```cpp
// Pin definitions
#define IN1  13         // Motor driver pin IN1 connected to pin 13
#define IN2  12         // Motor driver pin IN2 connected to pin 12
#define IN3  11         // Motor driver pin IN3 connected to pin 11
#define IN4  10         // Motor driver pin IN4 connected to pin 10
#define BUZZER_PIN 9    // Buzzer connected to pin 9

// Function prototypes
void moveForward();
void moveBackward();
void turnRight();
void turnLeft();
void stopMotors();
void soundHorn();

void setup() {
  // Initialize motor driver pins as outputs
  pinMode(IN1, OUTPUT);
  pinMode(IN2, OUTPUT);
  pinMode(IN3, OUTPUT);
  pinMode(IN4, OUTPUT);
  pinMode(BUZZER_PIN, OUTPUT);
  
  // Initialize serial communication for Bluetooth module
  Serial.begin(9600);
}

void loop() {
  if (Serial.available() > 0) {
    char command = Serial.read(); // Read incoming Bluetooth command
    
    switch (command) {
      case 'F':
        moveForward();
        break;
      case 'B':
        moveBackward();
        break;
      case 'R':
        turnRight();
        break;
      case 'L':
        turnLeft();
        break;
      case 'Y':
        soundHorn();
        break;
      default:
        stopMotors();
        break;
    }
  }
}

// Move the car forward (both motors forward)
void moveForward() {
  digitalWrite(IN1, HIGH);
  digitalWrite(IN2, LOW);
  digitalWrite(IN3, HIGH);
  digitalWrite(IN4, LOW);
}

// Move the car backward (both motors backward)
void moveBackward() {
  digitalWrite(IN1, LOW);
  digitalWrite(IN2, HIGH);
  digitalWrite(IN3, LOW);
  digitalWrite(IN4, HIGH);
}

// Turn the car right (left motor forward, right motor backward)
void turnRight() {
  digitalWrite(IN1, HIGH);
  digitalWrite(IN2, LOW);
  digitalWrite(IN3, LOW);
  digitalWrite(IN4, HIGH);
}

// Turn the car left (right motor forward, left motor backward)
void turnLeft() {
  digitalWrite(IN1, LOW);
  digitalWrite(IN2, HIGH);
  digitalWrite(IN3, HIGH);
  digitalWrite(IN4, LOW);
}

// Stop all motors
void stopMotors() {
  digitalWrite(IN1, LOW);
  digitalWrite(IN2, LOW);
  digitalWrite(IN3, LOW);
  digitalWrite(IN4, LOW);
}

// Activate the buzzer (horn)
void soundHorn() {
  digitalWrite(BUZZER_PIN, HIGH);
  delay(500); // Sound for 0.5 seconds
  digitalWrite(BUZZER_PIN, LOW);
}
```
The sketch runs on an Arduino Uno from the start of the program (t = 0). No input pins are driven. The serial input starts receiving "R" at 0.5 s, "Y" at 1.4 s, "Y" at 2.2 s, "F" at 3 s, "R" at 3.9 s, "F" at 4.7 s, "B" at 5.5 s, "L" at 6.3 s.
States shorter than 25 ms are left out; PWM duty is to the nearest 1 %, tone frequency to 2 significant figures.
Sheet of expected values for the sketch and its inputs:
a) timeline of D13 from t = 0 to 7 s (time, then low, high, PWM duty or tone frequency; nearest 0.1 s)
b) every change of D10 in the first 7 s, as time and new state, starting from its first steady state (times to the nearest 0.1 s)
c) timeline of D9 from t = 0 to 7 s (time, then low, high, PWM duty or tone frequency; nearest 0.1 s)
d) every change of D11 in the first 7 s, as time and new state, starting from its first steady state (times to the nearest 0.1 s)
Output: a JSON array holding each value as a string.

["0 s low; 0.5 s high; 5.5 s low", "0 s low; 0.5 s high; 3 s low; 3.9 s high; 4.7 s low; 5.5 s high; 6.3 s low", "0 s low; 1.4 s high; 1.9 s low; 2.2 s high; 2.7 s low", "0 s low; 3 s high; 3.9 s low; 4.7 s high; 5.5 s low; 6.3 s high"]
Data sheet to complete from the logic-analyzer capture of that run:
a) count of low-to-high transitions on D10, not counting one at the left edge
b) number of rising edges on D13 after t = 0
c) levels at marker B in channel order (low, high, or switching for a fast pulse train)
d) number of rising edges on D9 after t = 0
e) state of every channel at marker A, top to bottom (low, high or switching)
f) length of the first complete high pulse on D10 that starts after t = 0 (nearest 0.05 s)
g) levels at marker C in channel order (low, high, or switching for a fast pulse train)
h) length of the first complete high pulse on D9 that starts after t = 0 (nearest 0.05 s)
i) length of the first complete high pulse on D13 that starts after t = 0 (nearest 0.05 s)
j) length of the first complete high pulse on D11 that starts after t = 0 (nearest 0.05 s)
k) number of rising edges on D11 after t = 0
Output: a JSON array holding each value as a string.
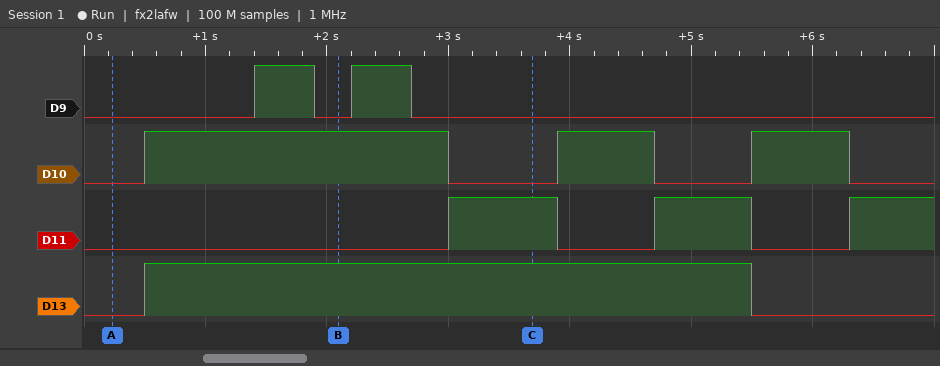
["3", "1", "D9 low, D10 high, D11 low, D13 high", "2", "D9 low, D10 low, D11 low, D13 low", "2.50 s", "D9 low, D10 low, D11 high, D13 high", "0.50 s", "5.00 s", "0.90 s", "3"]
